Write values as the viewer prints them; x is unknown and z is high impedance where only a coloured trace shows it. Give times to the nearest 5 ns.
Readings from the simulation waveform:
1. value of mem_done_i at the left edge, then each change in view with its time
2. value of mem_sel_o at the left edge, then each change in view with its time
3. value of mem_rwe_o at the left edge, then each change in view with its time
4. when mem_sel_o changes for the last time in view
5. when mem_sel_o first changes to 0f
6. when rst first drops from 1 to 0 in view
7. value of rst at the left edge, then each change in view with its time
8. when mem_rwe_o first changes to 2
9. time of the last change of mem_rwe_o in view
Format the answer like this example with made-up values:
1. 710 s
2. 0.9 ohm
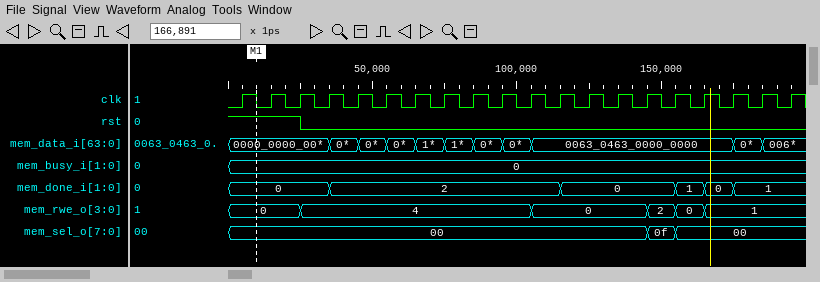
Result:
1. 0, 2 at 35 ns, 0 at 115 ns, 1 at 155 ns, 0 at 165 ns, 1 at 175 ns
2. 00, 0f at 145 ns, 00 at 155 ns
3. 0, 4 at 25 ns, 0 at 105 ns, 2 at 145 ns, 0 at 155 ns, 1 at 165 ns
4. 155 ns
5. 145 ns
6. 25 ns
7. 1, 0 at 25 ns
8. 145 ns
9. 165 ns
